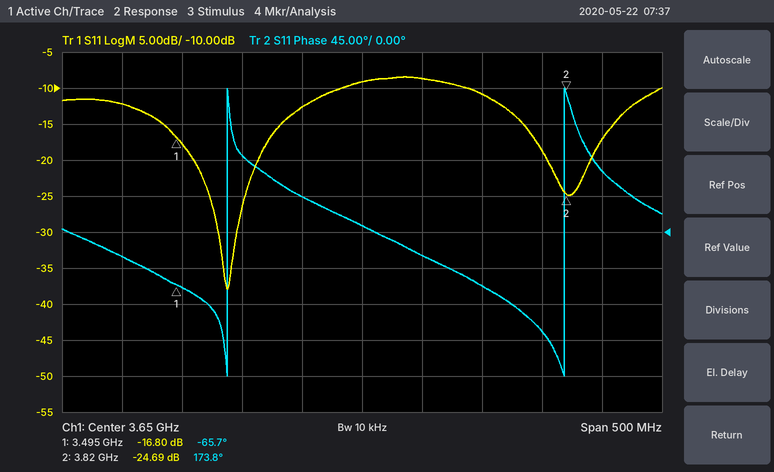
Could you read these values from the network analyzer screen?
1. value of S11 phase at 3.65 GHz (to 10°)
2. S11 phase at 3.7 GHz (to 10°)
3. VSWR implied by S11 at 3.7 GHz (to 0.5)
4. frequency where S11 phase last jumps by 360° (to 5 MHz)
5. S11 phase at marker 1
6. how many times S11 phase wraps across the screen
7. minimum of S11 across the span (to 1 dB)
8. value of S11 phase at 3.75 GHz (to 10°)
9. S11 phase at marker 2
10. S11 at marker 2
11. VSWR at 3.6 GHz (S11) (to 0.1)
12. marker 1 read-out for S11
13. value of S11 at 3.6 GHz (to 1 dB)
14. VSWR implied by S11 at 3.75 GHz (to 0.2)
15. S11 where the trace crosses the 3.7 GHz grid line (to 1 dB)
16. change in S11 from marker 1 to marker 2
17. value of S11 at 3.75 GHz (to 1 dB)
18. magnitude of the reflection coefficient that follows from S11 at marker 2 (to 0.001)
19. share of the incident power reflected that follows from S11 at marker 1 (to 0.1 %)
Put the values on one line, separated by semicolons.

10°; -30°; 2.0; 3.820 GHz; -65.7°; 2; -38 dB; -70°; 173.8°; -24.69 dB; 1.6; -16.80 dB; -13 dB; 1.8; -9 dB; -7.89 dB; -11 dB; 0.058; 2.1 %
